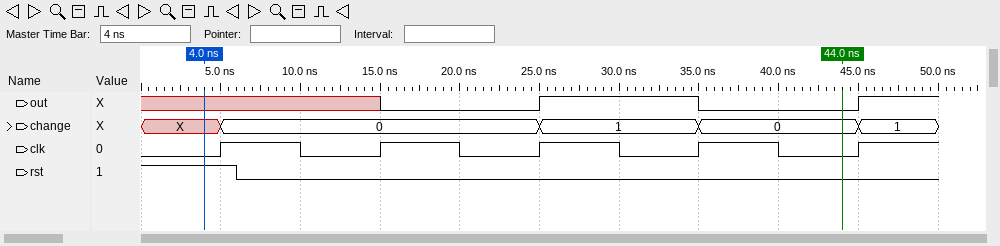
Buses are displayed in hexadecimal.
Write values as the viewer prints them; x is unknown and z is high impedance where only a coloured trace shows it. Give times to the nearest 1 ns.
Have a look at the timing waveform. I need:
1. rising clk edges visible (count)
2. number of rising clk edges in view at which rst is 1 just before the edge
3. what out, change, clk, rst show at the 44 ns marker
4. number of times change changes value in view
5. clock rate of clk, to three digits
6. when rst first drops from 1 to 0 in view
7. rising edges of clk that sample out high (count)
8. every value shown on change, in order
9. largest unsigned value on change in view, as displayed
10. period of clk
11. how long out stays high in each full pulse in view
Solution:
5
1
out=0, change=0, clk=0, rst=0
4
100 MHz
6 ns
1
X, 0, 1, 0, 1
1
10 ns
10 ns
